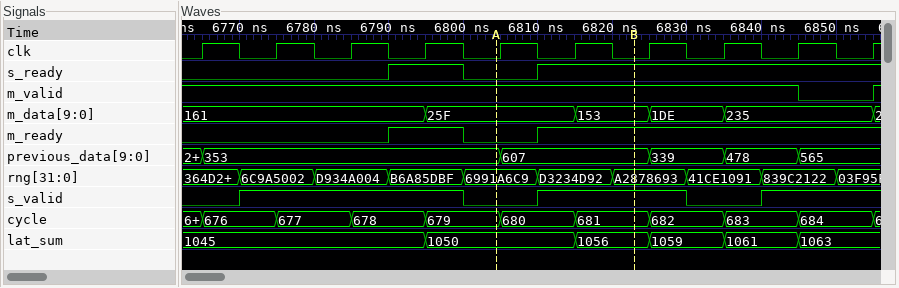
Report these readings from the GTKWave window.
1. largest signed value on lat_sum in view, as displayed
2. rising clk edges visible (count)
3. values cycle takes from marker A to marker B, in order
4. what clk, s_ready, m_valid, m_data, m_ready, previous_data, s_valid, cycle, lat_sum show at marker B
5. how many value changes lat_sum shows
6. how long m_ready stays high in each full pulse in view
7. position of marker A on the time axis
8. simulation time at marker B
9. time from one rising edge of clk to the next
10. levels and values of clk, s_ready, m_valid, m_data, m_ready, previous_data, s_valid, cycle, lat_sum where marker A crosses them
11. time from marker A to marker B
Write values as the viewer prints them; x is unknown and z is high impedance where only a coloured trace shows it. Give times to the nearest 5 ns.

1063
10
679, 680, 681
clk=0, s_ready=1, m_valid=1, m_data=153, m_ready=1, previous_data=607, s_valid=1, cycle=681, lat_sum=1056
5
10 ns
6805 ns
6825 ns
10 ns
clk=0, s_ready=0, m_valid=1, m_data=25F, m_ready=0, previous_data=353, s_valid=0, cycle=679, lat_sum=1050
20 ns
